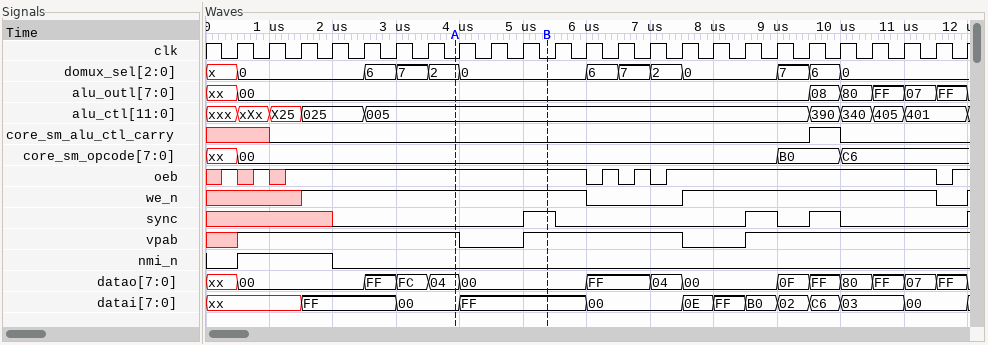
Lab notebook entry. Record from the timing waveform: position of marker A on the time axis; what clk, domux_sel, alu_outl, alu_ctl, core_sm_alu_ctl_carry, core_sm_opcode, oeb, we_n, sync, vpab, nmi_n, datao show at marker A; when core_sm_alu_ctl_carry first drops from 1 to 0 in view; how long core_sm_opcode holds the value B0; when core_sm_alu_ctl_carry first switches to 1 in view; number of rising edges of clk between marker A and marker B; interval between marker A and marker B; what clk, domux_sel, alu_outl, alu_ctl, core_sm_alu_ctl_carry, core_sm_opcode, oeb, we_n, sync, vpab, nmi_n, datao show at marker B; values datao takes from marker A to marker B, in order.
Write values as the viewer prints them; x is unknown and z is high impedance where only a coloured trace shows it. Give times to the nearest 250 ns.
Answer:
4000 ns
clk=0, domux_sel=2, alu_outl=00, alu_ctl=005, core_sm_alu_ctl_carry=0, core_sm_opcode=00, oeb=1, we_n=1, sync=0, vpab=1, nmi_n=0, datao=04
10000 ns
1000 ns
9500 ns
3
1500 ns
clk=0, domux_sel=0, alu_outl=00, alu_ctl=005, core_sm_alu_ctl_carry=0, core_sm_opcode=00, oeb=1, we_n=1, sync=1, vpab=1, nmi_n=0, datao=00
04, 00
